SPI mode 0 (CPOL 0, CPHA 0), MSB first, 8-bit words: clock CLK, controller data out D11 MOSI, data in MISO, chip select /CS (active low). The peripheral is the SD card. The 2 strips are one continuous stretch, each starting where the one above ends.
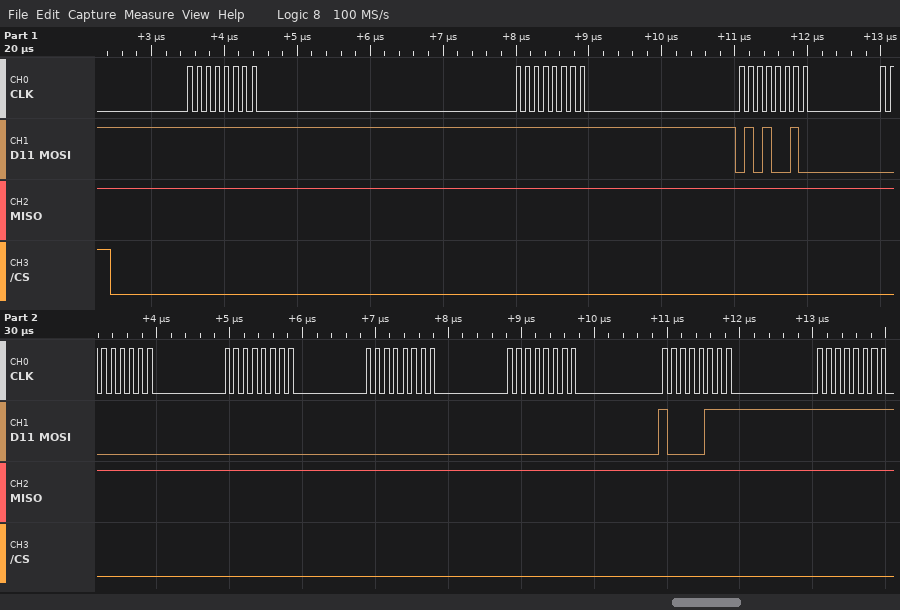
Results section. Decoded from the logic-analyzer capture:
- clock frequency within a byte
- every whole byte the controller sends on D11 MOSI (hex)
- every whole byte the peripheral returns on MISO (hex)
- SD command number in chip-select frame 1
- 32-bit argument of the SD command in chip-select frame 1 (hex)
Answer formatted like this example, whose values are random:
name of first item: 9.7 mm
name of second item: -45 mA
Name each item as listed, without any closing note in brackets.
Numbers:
clock frequency within a byte: 8 MHz
every whole byte the controller sends on D11 MOSI: FF FF 52 00 00 00 00 87 FF
every whole byte the peripheral returns on MISO: FF FF FF FF FF FF FF FF FF
SD command number in chip-select frame 1: CMD18
32-bit argument of the SD command in chip-select frame 1: 0x00000000
